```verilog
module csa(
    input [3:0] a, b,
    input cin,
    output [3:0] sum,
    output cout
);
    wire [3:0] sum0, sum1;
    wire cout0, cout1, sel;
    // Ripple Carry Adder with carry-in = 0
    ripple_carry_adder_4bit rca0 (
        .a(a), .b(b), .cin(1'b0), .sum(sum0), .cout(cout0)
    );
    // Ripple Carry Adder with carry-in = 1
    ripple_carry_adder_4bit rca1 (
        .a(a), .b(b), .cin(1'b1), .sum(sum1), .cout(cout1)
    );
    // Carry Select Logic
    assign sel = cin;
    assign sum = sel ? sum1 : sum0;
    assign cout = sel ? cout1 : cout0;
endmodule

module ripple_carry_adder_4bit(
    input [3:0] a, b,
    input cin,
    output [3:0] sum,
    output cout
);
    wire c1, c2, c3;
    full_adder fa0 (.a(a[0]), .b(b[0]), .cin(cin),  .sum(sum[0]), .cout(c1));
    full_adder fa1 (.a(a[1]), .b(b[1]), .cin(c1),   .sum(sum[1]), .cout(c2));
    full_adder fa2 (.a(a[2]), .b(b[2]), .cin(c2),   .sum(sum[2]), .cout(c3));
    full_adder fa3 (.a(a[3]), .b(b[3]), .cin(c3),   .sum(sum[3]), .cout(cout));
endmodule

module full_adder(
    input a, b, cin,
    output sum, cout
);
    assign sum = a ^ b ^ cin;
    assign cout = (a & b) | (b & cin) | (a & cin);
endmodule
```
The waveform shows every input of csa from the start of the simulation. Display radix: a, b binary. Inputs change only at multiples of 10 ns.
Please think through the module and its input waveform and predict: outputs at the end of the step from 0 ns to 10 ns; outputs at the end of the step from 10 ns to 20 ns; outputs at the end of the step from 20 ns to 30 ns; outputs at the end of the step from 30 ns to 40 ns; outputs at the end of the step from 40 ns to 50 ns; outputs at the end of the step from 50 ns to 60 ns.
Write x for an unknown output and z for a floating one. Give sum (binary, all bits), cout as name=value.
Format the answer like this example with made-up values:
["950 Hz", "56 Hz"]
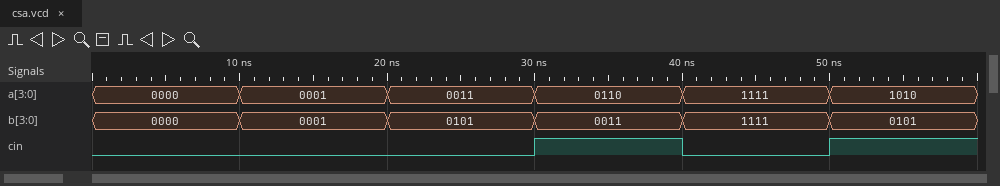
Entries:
["sum=0000, cout=0", "sum=0010, cout=0", "sum=1000, cout=0", "sum=1010, cout=0", "sum=1110, cout=1", "sum=0000, cout=1"]
